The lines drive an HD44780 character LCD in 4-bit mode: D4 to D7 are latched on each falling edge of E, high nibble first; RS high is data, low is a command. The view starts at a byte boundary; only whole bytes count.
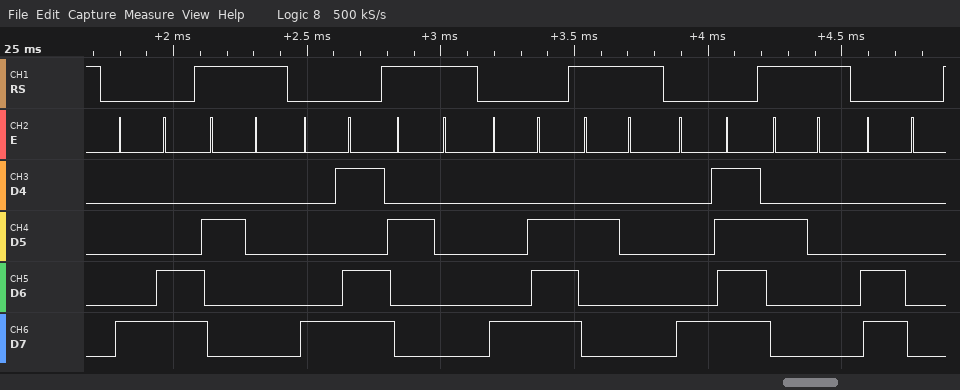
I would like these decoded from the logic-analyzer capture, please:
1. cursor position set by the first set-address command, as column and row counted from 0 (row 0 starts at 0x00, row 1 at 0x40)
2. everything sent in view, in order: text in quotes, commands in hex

column 12, row 0
0x8C " " 0x8D " " 0x8E " " 0x8F " " 0xC0
